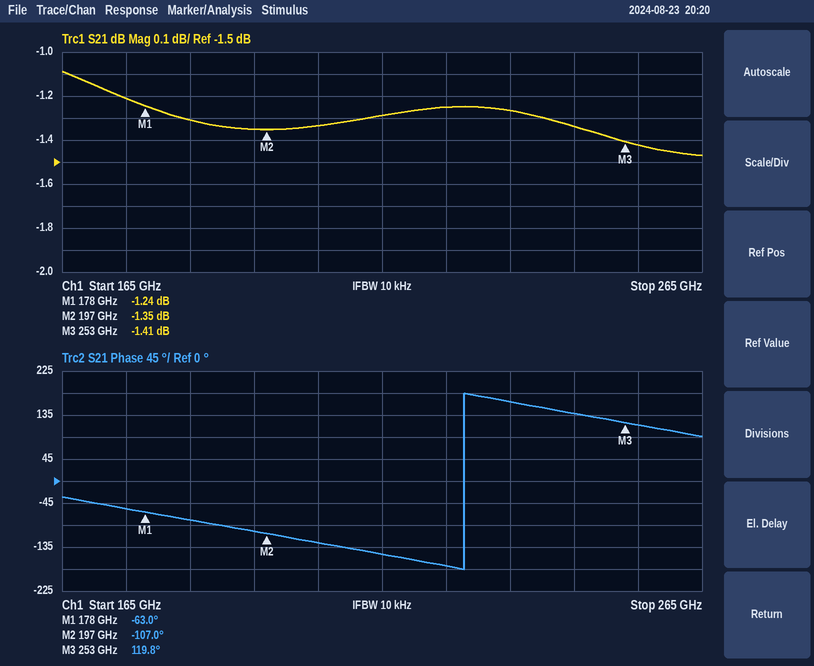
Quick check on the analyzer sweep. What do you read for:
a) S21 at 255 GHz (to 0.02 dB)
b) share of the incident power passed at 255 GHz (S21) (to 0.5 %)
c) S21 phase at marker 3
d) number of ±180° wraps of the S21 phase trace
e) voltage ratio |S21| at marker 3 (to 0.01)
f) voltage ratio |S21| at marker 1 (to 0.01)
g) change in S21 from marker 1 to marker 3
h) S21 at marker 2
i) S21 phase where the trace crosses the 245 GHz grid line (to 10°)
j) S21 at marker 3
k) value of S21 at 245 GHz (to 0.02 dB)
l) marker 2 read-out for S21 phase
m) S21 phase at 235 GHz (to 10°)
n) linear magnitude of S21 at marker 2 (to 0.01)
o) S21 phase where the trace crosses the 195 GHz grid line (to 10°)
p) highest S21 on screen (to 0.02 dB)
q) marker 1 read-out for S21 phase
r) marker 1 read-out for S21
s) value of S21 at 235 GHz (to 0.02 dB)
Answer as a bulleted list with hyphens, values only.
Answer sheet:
- -1.42 dB
- 72.0 %
- 119.8°
- 1
- 0.85
- 0.87
- -0.17 dB
- -1.35 dB
- 140°
- -1.41 dB
- -1.34 dB
- -107.0°
- 160°
- 0.86
- -100°
- -1.08 dB
- -63.0°
- -1.24 dB
- -1.26 dB
